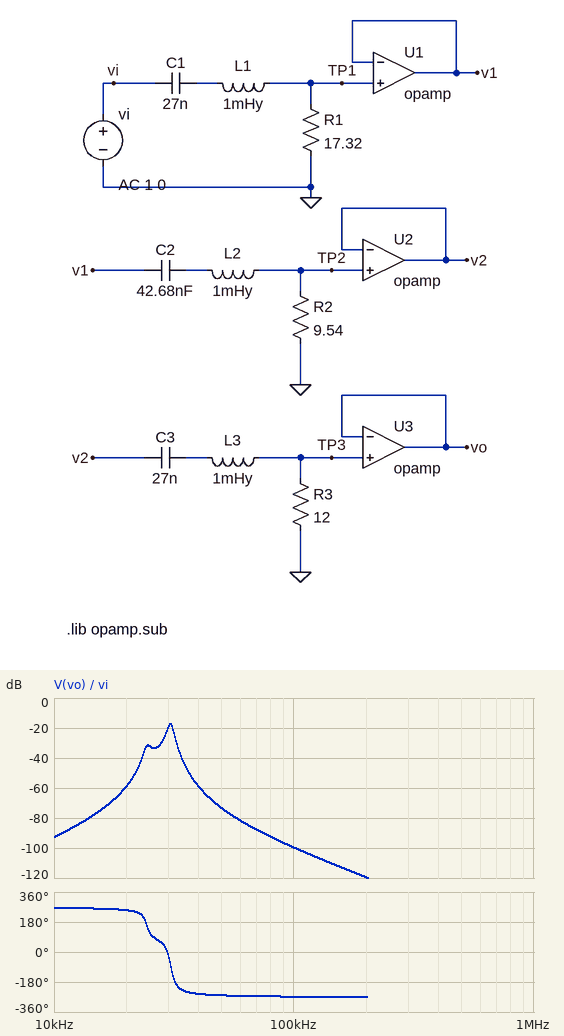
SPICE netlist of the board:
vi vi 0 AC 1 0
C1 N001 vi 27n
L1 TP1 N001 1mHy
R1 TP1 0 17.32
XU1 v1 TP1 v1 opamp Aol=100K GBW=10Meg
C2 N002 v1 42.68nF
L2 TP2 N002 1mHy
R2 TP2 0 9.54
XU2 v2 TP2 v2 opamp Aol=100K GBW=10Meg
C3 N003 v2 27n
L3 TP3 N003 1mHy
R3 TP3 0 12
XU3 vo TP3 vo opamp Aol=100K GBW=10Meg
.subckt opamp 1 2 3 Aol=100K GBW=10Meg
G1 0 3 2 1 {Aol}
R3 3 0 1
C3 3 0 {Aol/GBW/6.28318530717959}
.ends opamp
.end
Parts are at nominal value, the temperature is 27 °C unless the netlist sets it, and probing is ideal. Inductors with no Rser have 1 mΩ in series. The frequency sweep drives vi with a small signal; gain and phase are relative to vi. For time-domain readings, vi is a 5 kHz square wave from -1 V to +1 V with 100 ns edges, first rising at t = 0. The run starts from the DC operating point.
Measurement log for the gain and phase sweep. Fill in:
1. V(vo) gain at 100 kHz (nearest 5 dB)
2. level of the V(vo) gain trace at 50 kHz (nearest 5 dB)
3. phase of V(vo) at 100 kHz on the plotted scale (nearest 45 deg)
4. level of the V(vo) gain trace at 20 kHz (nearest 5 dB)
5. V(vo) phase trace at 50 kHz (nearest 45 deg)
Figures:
-100 dB
-75 dB
-270 deg
-60 dB
-270 deg
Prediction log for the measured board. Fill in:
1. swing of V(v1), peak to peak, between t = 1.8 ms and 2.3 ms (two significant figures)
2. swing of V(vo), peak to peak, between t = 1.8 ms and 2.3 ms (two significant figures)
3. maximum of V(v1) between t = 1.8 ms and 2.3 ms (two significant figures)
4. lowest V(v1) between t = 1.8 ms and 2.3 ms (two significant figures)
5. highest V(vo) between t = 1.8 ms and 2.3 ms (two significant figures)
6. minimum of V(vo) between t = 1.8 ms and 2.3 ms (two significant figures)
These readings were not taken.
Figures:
240 mV
15 mV
120 mV
-120 mV
7.4 mV
-7.4 mV
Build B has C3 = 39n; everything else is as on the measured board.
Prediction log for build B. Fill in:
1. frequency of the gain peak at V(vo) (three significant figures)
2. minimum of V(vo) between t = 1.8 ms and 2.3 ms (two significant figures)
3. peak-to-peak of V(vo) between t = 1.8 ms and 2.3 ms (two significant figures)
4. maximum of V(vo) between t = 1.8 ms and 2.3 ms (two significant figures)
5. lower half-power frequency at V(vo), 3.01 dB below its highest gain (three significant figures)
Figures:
25.0 kHz
-38 mV
76 mV
38 mV
24.2 kHz
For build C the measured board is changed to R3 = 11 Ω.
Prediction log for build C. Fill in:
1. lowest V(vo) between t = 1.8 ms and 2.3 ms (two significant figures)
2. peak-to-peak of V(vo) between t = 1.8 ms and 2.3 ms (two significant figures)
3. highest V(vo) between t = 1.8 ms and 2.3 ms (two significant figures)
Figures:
-6.8 mV
14 mV
6.8 mV
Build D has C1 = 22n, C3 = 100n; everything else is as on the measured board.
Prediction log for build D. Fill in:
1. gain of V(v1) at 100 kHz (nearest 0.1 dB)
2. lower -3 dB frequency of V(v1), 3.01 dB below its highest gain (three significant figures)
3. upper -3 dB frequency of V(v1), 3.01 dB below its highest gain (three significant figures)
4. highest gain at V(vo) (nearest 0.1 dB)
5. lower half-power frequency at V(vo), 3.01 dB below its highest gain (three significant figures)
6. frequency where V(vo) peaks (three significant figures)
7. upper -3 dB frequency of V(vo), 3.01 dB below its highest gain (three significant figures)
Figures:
-30.1 dB
32.6 kHz
35.3 kHz
-35.8 dB
23.6 kHz
24.4 kHz
25.2 kHz
